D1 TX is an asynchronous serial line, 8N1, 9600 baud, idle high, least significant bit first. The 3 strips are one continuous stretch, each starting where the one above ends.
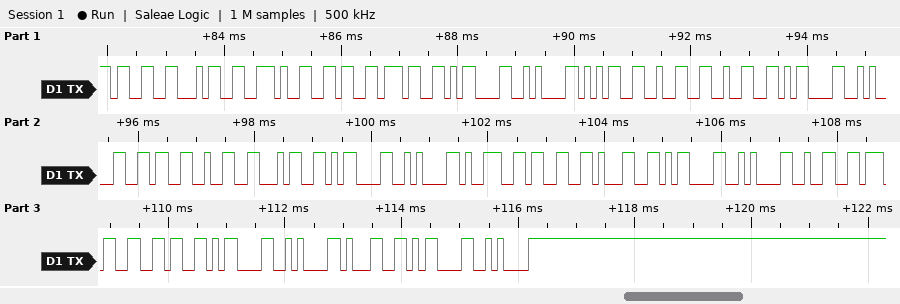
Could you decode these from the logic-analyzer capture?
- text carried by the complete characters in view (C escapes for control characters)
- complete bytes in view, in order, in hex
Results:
"34.67\r\n522\r\n624\r\n931\r\n276\r\n1\r\n"
33 34 2E 36 37 0D 0A 35 32 32 0D 0A 36 32 34 0D 0A 39 33 31 0D 0A 32 37 36 0D 0A 31 0D 0A
